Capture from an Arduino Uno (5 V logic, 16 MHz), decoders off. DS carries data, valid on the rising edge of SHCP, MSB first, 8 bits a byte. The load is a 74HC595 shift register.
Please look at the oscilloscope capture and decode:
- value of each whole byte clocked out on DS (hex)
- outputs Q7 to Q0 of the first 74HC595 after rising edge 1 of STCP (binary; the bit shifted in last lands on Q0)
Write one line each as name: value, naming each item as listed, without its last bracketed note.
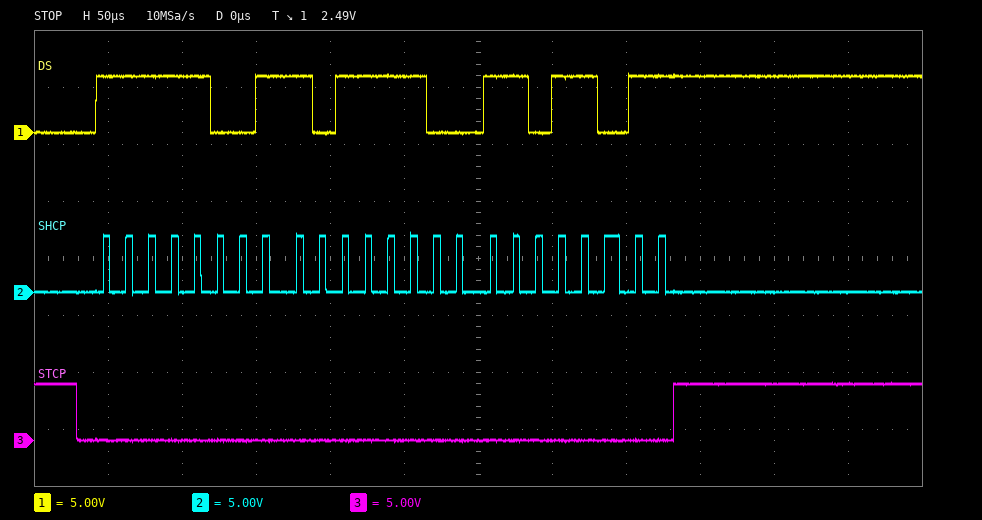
value of each whole byte clocked out on DS: 0xF9 0xBC 0xDB
outputs Q7 to Q0 of the first 74HC595 after rising edge 1 of STCP: 11011011
